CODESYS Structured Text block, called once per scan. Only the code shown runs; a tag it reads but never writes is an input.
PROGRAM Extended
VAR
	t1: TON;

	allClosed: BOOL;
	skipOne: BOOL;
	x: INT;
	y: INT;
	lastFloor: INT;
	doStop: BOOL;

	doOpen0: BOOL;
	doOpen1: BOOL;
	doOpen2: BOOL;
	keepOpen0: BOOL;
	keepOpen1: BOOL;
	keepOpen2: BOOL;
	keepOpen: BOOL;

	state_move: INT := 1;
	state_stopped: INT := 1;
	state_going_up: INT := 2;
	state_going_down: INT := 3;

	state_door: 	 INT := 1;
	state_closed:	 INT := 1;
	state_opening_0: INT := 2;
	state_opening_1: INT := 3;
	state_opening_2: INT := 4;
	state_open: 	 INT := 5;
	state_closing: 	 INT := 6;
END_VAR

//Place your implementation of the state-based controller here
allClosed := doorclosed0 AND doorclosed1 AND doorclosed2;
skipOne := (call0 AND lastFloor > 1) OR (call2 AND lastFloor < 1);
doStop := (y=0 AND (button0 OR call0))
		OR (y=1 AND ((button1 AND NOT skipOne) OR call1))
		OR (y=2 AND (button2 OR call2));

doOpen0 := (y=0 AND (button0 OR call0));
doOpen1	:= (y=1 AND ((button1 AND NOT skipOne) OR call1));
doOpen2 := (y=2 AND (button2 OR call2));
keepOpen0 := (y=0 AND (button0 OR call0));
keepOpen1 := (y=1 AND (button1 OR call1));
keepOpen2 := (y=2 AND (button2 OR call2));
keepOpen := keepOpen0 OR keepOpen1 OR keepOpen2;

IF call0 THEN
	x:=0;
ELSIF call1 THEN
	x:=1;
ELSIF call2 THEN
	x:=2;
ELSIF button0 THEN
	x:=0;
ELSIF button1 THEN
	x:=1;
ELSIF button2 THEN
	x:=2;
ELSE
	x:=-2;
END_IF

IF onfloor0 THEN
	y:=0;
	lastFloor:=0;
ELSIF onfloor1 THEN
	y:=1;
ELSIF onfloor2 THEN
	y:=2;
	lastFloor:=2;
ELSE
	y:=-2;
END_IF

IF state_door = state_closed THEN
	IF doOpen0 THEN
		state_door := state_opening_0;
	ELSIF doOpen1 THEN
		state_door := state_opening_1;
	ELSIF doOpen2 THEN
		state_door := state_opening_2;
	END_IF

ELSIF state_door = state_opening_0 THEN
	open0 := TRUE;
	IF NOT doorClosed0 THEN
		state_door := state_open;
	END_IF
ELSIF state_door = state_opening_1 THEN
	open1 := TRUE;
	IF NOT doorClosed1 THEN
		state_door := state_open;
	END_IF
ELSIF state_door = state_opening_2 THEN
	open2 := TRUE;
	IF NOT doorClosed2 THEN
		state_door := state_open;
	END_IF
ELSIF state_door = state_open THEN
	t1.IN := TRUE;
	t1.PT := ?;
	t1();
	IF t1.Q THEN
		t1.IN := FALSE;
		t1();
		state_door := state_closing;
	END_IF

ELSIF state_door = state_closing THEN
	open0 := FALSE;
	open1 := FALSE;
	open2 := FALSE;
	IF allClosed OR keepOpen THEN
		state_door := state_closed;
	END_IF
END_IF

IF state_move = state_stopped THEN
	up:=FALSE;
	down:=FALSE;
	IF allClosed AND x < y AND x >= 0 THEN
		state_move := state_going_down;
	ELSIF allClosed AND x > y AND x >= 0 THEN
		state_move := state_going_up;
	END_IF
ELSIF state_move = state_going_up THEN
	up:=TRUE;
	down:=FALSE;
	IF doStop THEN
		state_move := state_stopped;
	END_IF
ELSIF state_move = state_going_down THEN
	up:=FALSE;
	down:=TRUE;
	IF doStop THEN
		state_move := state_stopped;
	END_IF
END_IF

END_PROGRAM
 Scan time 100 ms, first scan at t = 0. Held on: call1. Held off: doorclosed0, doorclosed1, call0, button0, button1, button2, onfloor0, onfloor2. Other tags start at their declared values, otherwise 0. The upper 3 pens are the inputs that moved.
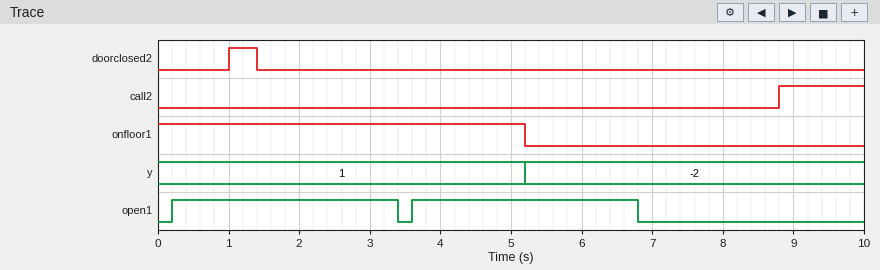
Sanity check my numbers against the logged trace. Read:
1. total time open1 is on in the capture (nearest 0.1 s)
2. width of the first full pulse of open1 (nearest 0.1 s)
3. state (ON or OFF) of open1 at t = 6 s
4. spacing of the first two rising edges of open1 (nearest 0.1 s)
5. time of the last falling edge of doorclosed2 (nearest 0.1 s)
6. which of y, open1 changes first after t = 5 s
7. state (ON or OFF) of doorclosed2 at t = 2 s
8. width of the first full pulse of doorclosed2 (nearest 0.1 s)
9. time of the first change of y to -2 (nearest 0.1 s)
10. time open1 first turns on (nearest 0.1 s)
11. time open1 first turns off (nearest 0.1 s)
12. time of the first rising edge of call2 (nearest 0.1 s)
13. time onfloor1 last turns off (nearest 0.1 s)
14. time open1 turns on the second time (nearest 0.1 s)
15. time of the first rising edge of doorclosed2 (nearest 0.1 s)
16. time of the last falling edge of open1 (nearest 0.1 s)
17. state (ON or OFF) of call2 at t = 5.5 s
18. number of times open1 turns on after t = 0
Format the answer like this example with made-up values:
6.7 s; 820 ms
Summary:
6.4 s; 3.2 s; ON; 3.4 s; 1.4 s; y; OFF; 0.4 s; 5.2 s; 0.2 s; 3.4 s; 8.8 s; 5.2 s; 3.6 s; 1.0 s; 6.8 s; OFF; 2
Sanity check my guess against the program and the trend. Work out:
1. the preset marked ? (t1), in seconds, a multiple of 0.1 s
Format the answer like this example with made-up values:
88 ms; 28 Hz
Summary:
3.0 s
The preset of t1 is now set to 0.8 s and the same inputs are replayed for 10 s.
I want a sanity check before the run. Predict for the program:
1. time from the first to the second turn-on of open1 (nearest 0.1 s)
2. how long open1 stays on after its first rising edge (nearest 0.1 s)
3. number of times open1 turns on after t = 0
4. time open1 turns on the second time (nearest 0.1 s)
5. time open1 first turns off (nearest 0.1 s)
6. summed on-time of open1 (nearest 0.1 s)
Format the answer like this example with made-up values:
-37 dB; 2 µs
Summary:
1.2 s; 1.0 s; 5; 1.4 s; 1.2 s; 5.0 s
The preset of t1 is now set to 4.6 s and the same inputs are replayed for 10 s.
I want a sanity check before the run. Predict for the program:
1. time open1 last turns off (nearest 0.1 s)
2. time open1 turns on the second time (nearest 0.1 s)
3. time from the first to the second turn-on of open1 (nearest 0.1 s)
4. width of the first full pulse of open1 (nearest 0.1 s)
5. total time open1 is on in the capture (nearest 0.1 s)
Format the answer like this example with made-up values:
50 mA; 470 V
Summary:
5.0 s; 5.2 s; 5.0 s; 4.8 s; 9.6 s
